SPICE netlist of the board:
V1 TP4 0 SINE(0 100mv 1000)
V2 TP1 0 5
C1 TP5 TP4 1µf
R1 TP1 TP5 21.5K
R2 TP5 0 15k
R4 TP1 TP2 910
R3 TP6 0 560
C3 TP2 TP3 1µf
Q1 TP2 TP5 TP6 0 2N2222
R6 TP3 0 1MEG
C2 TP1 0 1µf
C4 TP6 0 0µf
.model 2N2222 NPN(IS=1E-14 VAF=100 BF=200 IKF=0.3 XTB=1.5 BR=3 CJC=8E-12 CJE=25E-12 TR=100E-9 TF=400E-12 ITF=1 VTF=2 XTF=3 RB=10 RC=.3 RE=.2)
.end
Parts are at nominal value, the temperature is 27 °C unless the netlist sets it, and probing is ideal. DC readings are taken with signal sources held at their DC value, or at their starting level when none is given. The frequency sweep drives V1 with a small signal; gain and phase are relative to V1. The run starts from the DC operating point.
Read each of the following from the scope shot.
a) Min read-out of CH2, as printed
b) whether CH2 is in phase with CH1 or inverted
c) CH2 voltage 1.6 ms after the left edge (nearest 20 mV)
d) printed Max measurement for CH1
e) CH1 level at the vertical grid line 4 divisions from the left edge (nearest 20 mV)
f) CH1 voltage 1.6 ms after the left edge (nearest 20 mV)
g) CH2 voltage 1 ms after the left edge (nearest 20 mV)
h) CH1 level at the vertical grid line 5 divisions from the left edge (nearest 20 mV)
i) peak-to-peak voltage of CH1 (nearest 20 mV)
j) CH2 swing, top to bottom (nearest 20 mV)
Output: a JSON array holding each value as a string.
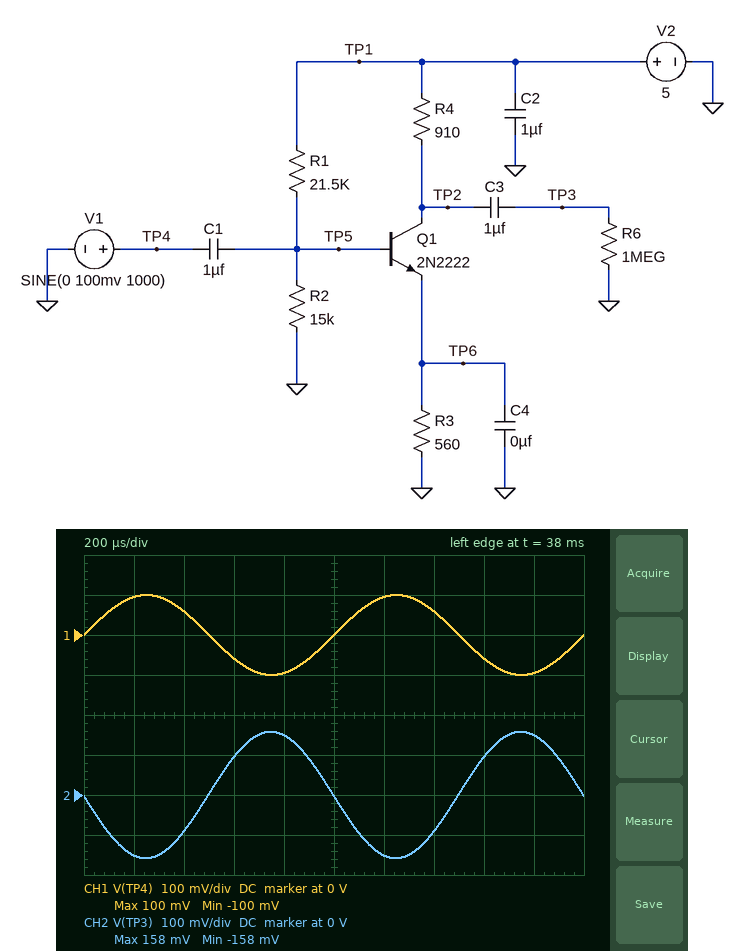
["-158 mV", "inverted", "100 mV", "100 mV", "-100 mV", "-60 mV", "0 V", "0 V", "200 mV", "320 mV"]
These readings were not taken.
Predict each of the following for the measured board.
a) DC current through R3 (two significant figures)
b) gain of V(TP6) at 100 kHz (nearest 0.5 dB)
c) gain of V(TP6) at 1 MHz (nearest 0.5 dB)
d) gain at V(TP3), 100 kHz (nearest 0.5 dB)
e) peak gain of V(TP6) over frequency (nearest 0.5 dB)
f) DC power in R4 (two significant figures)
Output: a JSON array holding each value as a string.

["2.3 mA", "0 dB", "0 dB", "4.0 dB", "0 dB", "4.7 mW"]
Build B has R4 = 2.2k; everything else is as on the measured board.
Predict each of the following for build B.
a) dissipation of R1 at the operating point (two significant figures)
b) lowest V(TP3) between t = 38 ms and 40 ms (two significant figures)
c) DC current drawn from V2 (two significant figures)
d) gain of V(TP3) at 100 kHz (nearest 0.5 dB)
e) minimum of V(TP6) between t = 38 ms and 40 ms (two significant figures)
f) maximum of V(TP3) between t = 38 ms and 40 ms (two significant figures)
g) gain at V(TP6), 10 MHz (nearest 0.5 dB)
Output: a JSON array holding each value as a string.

["510 µW", "-7.1 mV", "1.9 mA", "-12.0 dB", "880 mV", "450 mV", "-0.5 dB"]
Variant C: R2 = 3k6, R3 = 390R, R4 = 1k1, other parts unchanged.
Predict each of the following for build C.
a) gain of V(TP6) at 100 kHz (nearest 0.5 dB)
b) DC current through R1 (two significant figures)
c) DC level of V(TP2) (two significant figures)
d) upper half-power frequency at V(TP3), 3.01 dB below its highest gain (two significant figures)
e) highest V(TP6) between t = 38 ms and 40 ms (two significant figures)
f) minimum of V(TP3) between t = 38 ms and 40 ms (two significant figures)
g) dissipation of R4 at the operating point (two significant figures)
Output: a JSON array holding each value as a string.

["-2.0 dB", "200 µA", "4.7 V", "45 MHz", "180 mV", "-230 mV", "66 µW"]
